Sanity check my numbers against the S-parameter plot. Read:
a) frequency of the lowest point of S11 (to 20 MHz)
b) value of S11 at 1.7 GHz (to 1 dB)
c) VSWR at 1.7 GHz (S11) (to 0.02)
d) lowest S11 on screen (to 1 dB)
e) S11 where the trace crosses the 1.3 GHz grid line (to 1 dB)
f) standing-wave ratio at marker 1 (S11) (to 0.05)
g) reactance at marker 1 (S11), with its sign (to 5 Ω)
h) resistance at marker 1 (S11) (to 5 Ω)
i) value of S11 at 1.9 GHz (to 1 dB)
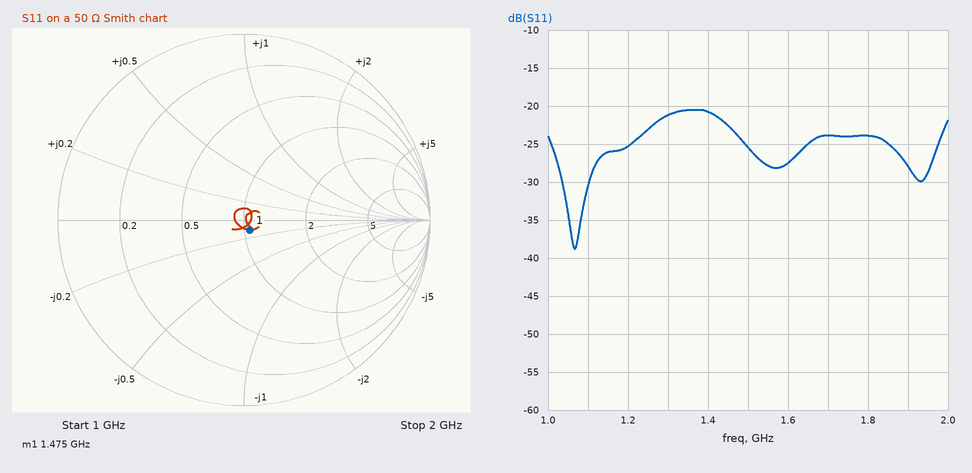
1.06 GHz
-24 dB
1.14
-39 dB
-21 dB
1.15
-5 Ω
55 Ω
-28 dB
